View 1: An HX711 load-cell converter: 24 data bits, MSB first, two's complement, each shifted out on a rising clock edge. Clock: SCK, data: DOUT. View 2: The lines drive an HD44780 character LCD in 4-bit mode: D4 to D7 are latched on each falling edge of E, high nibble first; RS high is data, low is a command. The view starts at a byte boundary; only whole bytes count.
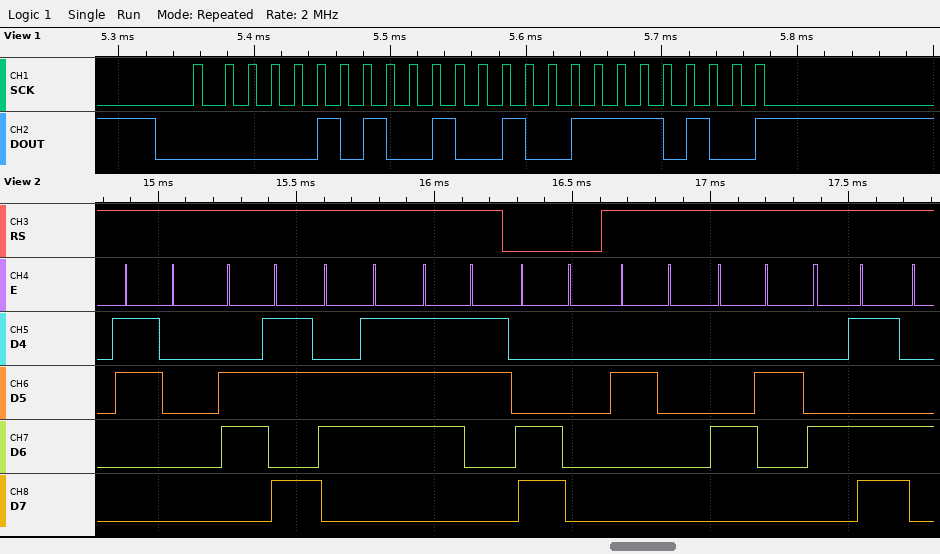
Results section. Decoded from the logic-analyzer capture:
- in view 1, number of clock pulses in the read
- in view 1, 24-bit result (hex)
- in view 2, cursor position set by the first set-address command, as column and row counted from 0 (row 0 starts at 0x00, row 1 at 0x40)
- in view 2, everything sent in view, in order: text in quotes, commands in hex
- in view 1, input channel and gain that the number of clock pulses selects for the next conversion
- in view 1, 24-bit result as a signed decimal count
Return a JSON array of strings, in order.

["25", "0x0524F4", "column 0, row 1", "\"0kgs\" 0xC0 \" BM\"", "channel A, gain 128", "337140"]
